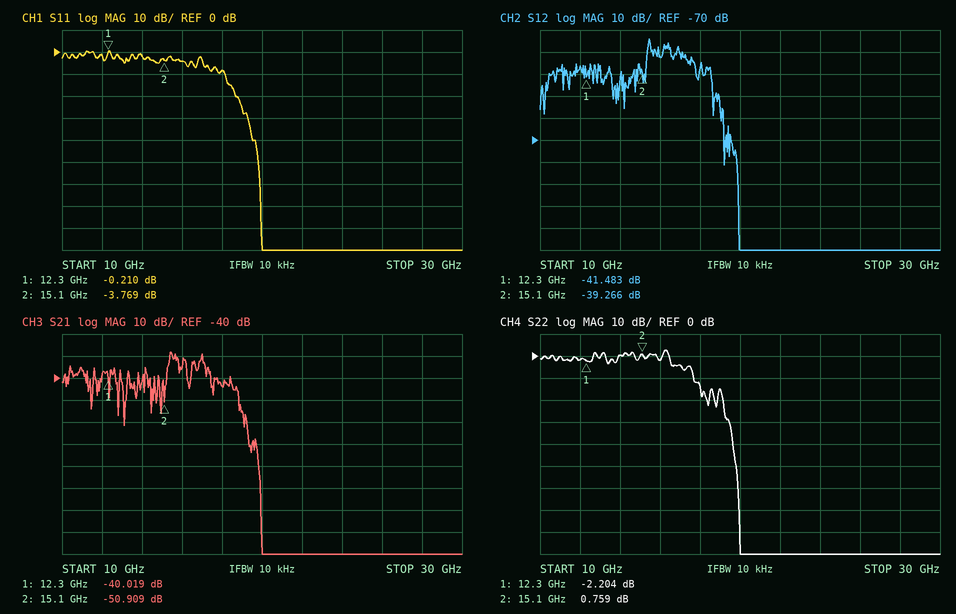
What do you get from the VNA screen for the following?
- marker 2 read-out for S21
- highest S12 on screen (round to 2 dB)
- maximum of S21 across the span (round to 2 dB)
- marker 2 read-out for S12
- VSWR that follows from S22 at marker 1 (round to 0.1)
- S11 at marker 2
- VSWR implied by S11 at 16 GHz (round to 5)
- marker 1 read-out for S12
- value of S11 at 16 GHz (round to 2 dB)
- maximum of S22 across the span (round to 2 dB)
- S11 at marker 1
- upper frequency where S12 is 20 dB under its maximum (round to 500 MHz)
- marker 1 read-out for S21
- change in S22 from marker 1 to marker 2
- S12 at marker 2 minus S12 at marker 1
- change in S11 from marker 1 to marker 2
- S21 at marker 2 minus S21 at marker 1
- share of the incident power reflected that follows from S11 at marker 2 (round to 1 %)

-50.909 dB
-24 dB
-28 dB
-39.266 dB
7.9
-3.769 dB
5
-41.483 dB
-4 dB
2 dB
-0.210 dB
18.5 GHz
-40.019 dB
2.963 dB
2.217 dB
-3.559 dB
-10.890 dB
42 %
